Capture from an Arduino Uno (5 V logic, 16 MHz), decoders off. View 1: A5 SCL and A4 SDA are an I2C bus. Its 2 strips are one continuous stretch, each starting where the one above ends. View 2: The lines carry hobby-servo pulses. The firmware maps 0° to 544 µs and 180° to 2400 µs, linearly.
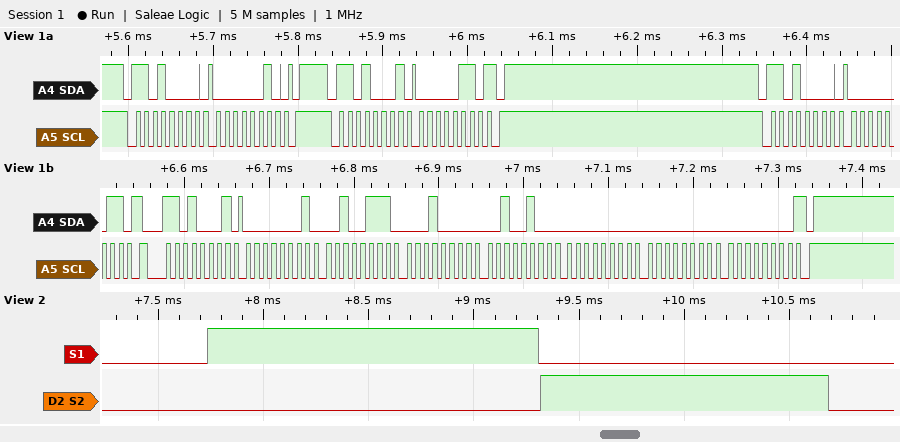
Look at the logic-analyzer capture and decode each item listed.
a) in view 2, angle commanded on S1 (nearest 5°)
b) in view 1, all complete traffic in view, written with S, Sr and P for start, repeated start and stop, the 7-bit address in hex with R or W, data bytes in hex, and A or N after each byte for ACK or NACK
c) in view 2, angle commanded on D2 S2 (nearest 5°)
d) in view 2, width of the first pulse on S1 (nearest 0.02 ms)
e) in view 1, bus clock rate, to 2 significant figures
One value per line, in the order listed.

100°
S 68W A 02 A P S 68R A 06 N P S 68W A 03 A Sr 68R A 01 A 27 A 10 A 24 A 00 A 00 A 00 N P
80°
1.58 ms
100 kHz
